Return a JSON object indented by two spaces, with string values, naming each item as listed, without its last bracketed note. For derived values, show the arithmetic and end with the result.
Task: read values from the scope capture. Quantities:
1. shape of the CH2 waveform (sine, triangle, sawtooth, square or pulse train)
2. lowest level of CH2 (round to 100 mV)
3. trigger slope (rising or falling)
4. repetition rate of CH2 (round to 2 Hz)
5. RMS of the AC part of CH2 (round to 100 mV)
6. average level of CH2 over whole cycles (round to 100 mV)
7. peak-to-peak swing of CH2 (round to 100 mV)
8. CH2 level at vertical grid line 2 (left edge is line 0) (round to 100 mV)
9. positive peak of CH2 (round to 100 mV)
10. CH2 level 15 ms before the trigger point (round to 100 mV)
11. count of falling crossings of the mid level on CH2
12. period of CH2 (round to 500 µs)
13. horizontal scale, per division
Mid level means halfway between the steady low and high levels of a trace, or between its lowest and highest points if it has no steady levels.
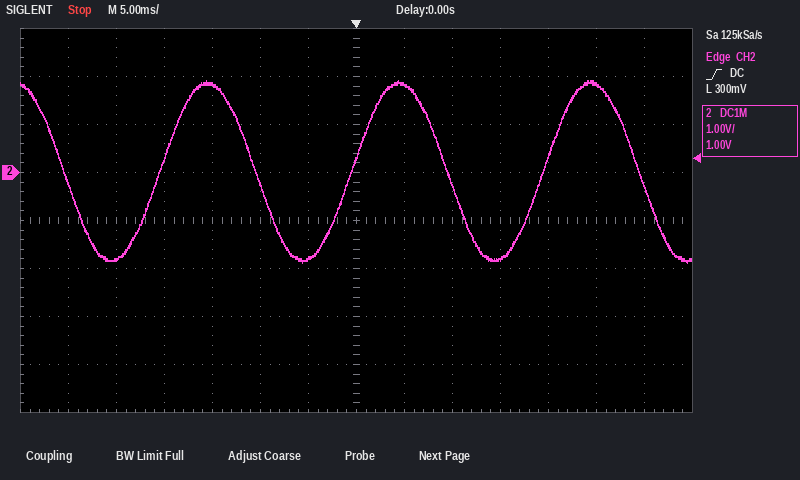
{
  "shape of the CH2 waveform": "sine",
  "lowest level of CH2": "-1.9 V",
  "trigger slope": "rising",
  "repetition rate of CH2": "1 / 20.0 ms ≈ 50 Hz",
  "RMS of the AC part of CH2": "3.8 V / (2√2) ≈ 1.3 V",
  "average level of CH2 over whole cycles": "(1.9 V + (-1.9 V)) / 2 ≈ 0.0 V",
  "peak-to-peak swing of CH2": "1.9 V − (-1.9 V) = 3.8 V",
  "CH2 level at vertical grid line 2 (left edge is line 0)": "-1.8 V",
  "positive peak of CH2": "1.9 V",
  "CH2 level 15 ms before the trigger point": "1.8 V",
  "count of falling crossings of the mid level on CH2": "4",
  "period of CH2": "20.0 ms",
  "horizontal scale, per division": "5 ms"
}
